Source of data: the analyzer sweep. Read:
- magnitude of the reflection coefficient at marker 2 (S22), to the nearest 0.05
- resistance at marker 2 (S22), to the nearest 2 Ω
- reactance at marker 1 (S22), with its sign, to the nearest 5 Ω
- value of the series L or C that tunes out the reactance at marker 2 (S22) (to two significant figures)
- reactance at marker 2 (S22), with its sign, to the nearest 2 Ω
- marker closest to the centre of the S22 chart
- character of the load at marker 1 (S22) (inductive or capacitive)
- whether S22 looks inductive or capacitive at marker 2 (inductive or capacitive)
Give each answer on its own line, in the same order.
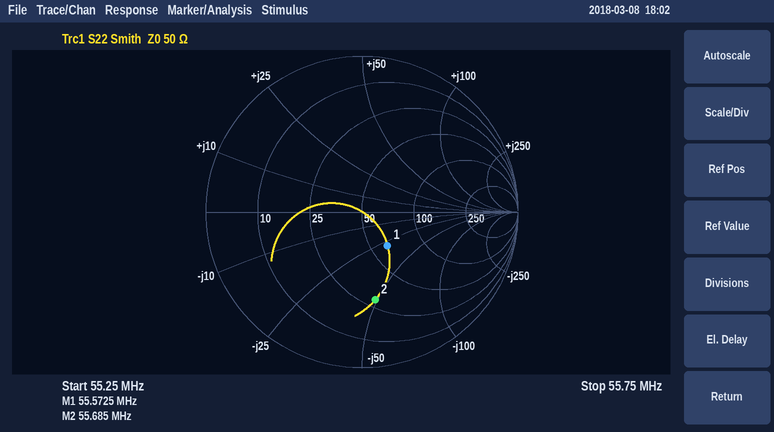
0.55
30 Ω
-30 Ω
140 nH
-48 Ω
marker 1
capacitive
capacitive
